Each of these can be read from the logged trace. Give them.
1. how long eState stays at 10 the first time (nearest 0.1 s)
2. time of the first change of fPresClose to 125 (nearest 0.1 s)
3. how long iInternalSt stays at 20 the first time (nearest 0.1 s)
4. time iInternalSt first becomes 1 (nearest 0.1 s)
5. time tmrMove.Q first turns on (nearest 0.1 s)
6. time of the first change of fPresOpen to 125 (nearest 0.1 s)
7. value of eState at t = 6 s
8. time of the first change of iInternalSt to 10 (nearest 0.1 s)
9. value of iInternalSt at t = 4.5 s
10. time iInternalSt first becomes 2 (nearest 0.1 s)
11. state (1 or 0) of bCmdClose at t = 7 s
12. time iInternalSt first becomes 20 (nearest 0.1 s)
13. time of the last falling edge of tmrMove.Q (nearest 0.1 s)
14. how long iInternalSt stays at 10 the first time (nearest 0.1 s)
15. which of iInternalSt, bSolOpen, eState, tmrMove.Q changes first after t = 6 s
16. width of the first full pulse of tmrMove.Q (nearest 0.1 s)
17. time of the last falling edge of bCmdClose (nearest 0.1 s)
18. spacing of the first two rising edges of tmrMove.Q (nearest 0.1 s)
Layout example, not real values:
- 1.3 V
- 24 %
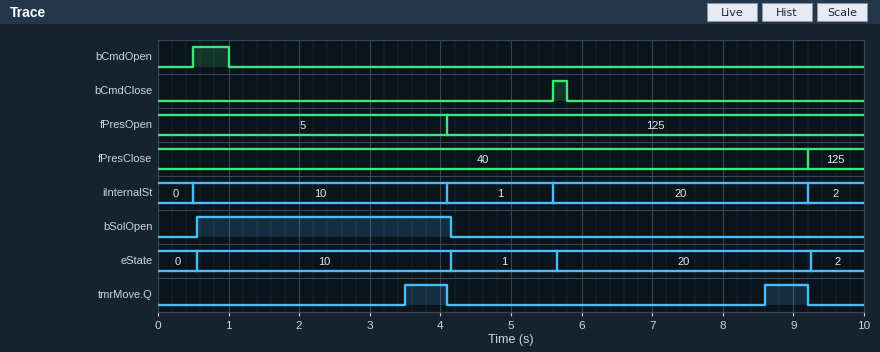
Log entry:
- 3.6 s
- 9.2 s
- 3.6 s
- 4.1 s
- 3.5 s
- 4.1 s
- 20
- 0.5 s
- 1
- 9.2 s
- 0
- 5.6 s
- 9.2 s
- 3.6 s
- tmrMove.Q
- 0.6 s
- 5.8 s
- 5.1 s
